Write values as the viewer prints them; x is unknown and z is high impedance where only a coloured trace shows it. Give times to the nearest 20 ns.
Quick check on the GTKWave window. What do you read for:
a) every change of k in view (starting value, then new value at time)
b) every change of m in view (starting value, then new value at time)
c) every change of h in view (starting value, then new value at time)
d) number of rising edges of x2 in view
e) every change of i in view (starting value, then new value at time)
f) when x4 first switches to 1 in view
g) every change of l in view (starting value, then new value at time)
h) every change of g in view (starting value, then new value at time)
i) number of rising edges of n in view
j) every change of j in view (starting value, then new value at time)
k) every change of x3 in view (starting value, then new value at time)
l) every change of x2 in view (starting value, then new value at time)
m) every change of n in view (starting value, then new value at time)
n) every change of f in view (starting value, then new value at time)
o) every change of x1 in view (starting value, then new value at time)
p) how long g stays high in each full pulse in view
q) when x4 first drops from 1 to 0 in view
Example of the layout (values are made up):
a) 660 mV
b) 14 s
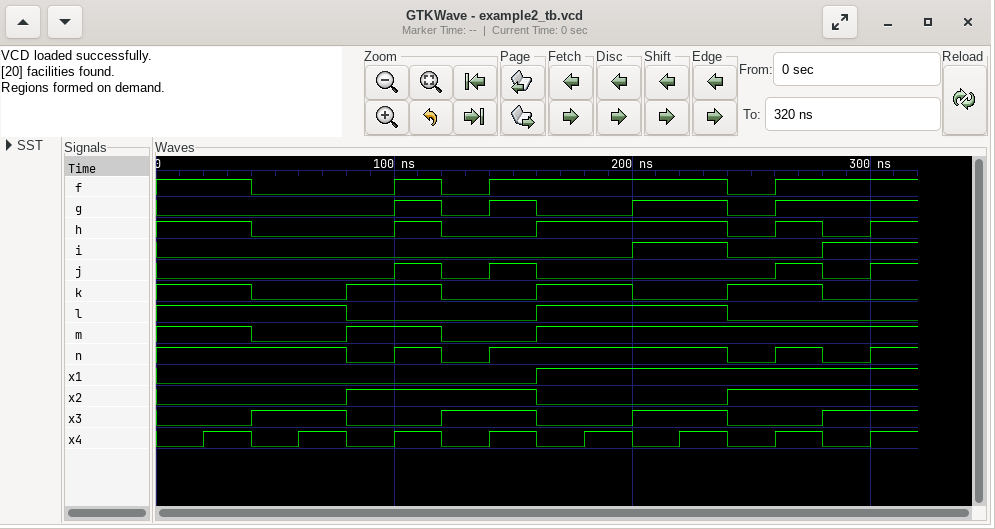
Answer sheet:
a) 1, 0 at 40 ns, 1 at 80 ns, 0 at 120 ns, 1 at 160 ns, 0 at 200 ns, 1 at 240 ns, 0 at 280 ns
b) 1, 0 at 40 ns, 1 at 80 ns, 0 at 120 ns, 1 at 160 ns
c) 1, 0 at 40 ns, 1 at 100 ns, 0 at 120 ns, 1 at 160 ns, 0 at 240 ns, 1 at 260 ns, 0 at 280 ns, 1 at 300 ns
d) 2
e) 0, 1 at 200 ns, 0 at 240 ns, 1 at 280 ns
f) 20 ns
g) 1, 0 at 80 ns, 1 at 160 ns, 0 at 240 ns
h) 0, 1 at 100 ns, 0 at 120 ns, 1 at 140 ns, 0 at 160 ns, 1 at 200 ns, 0 at 240 ns, 1 at 260 ns
i) 4
j) 0, 1 at 100 ns, 0 at 120 ns, 1 at 140 ns, 0 at 160 ns, 1 at 260 ns, 0 at 280 ns, 1 at 300 ns
k) 0, 1 at 40 ns, 0 at 80 ns, 1 at 120 ns, 0 at 160 ns, 1 at 200 ns, 0 at 240 ns, 1 at 280 ns
l) 0, 1 at 80 ns, 0 at 160 ns, 1 at 240 ns
m) 1, 0 at 80 ns, 1 at 100 ns, 0 at 120 ns, 1 at 140 ns, 0 at 240 ns, 1 at 260 ns, 0 at 280 ns, 1 at 300 ns
n) 1, 0 at 40 ns, 1 at 100 ns, 0 at 120 ns, 1 at 140 ns, 0 at 240 ns, 1 at 260 ns
o) 0, 1 at 160 ns
p) 20 ns, 20 ns, 40 ns
q) 40 ns
